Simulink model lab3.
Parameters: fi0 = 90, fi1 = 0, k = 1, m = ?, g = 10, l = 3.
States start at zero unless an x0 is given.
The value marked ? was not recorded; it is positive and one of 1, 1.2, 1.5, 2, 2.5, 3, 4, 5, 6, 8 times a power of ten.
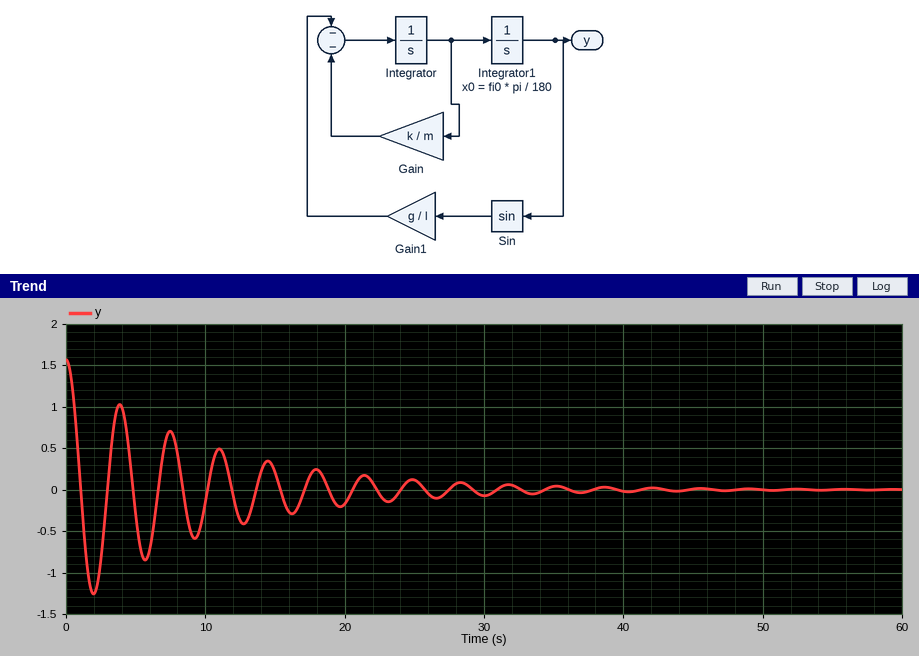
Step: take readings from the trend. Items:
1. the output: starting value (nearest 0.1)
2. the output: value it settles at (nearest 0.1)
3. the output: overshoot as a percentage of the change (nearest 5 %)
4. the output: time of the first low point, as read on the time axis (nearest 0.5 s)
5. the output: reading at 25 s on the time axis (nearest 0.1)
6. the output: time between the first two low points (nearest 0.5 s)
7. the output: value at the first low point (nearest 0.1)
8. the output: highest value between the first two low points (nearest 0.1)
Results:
1.6
0.0
80 %
2.0 s
0.1
3.5 s
-1.3
1.0
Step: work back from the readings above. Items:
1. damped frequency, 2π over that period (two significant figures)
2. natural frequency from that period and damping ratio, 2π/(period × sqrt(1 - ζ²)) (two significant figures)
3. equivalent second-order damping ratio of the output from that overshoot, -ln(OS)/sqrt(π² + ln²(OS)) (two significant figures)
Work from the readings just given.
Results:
1.8 rad/s
1.8 rad/s
0.071
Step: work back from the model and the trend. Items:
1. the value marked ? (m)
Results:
5
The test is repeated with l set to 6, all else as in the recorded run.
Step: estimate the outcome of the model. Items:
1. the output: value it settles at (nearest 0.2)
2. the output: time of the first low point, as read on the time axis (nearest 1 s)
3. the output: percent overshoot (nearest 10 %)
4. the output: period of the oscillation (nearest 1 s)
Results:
0.0
3 s
70 %
5 s
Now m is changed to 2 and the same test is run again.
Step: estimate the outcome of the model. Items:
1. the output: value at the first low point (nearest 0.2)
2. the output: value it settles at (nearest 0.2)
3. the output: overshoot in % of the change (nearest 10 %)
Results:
-1.0
0.0
60 %
